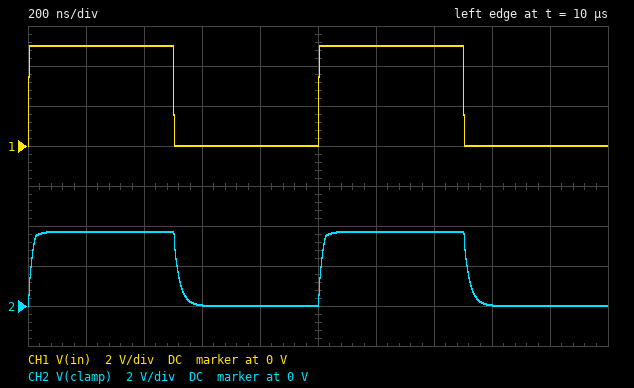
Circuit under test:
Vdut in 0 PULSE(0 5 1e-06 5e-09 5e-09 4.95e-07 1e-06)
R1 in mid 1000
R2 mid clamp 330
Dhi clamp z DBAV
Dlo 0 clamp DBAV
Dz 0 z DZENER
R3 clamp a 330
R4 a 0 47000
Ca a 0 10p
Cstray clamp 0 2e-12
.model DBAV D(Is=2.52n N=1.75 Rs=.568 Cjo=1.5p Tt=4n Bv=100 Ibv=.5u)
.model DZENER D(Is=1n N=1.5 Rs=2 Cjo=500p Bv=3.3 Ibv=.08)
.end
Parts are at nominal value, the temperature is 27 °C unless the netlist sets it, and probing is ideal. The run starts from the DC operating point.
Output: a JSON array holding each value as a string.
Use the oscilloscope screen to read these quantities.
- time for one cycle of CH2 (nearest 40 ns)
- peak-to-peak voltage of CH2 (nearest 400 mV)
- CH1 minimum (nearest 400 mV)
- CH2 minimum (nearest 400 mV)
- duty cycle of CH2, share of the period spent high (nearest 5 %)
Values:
["1.00 µs", "3.6 V", "0 V", "0 V", "50 %"]
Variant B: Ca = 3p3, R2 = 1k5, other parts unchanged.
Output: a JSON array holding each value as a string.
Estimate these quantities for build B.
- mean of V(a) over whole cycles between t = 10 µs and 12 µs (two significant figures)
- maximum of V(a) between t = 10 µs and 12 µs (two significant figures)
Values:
["1.8 V", "3.6 V"]
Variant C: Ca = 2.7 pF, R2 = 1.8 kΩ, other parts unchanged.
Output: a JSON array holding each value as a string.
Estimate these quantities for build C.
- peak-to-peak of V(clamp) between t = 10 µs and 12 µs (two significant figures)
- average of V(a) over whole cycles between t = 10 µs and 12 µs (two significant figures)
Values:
["3.6 V", "1.8 V"]
